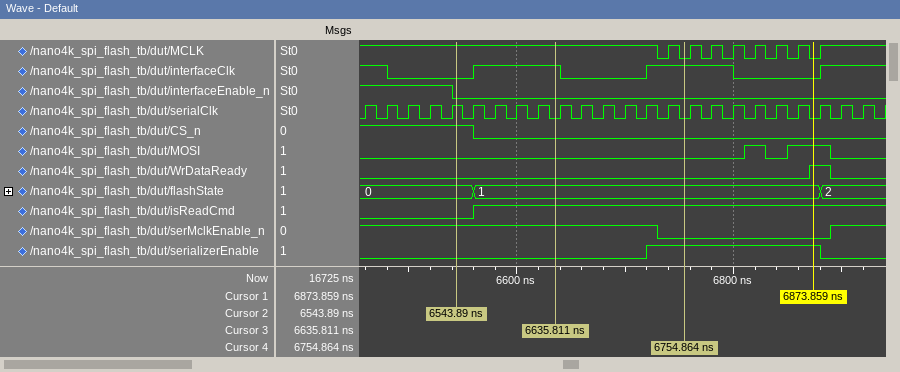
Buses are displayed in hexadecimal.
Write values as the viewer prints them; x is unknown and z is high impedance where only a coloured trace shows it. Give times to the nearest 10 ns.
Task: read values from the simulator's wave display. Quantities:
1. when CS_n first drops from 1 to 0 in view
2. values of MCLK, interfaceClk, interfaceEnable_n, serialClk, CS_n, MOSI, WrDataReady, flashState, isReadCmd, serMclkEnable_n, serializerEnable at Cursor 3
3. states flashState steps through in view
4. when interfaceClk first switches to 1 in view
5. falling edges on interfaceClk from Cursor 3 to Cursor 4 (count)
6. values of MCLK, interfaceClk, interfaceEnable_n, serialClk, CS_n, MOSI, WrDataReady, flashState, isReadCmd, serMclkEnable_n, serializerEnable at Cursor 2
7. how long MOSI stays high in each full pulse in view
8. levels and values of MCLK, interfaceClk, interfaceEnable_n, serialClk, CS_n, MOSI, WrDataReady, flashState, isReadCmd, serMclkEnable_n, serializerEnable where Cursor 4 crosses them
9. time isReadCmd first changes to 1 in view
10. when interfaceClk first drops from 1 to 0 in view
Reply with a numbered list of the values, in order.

1. 6560 ns
2. MCLK=1, interfaceClk=1, interfaceEnable_n=0, serialClk=0, CS_n=0, MOSI=0, WrDataReady=0, flashState=1, isReadCmd=1, serMclkEnable_n=1, serializerEnable=0
3. 0, 1, 2
4. 6560 ns
5. 1
6. MCLK=1, interfaceClk=0, interfaceEnable_n=0, serialClk=1, CS_n=1, MOSI=0, WrDataReady=0, flashState=0, isReadCmd=0, serMclkEnable_n=1, serializerEnable=0
7. 20 ns, 40 ns
8. MCLK=0, interfaceClk=1, interfaceEnable_n=0, serialClk=0, CS_n=0, MOSI=0, WrDataReady=0, flashState=1, isReadCmd=1, serMclkEnable_n=0, serializerEnable=1
9. 6560 ns
10. 6480 ns
